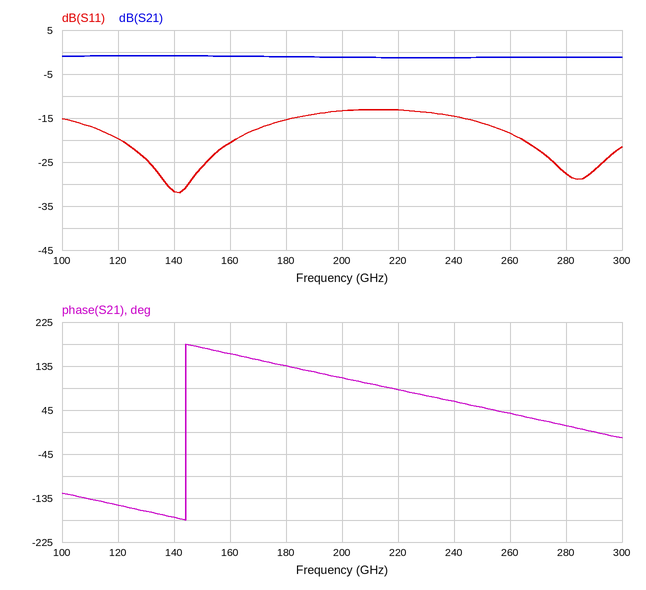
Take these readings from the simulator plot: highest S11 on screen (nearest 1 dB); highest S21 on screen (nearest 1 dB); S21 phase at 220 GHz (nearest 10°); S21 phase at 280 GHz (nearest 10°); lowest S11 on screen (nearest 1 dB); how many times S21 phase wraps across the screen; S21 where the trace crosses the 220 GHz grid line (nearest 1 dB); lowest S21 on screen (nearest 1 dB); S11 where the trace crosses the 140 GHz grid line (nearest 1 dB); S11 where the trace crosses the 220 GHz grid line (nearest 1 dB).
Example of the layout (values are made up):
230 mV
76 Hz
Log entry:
-13 dB
-1 dB
90°
10°
-32 dB
1
-1 dB
-1 dB
-32 dB
-13 dB
